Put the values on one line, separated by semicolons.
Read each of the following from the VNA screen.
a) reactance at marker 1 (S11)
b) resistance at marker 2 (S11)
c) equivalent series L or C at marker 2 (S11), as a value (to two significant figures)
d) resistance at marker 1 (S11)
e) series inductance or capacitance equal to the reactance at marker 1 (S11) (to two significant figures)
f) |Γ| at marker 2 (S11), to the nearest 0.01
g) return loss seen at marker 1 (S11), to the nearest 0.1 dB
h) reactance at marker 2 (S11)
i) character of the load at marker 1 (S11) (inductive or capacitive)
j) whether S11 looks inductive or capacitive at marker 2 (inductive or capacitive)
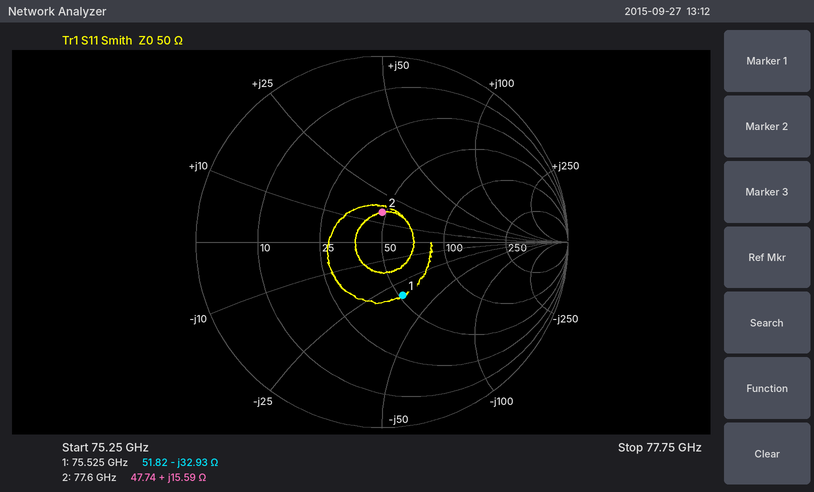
-32.93 Ω; 47.74 Ω; 32 pH; 51.82 Ω; 64 fF; 0.16; 10.2 dB; +15.59 Ω; capacitive; inductive
